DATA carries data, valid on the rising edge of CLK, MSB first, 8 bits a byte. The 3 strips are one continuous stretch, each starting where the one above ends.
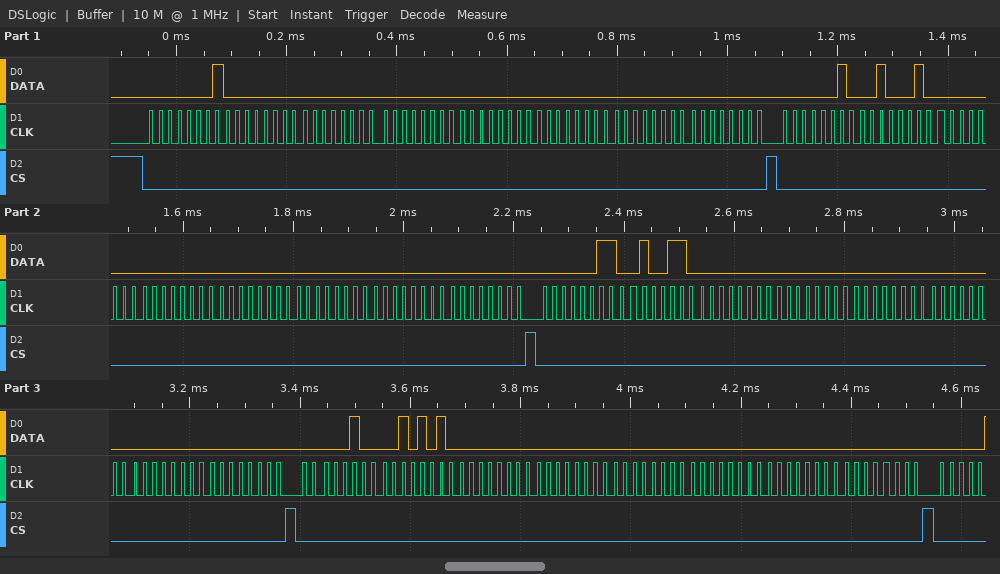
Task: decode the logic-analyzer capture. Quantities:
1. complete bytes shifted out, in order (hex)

01 00 00 00 00 00 00 00 02 22 00 00 00 00 00 00 03 26 00 00 00 00 00 00 04 2A 00 00 00 00 00 00
